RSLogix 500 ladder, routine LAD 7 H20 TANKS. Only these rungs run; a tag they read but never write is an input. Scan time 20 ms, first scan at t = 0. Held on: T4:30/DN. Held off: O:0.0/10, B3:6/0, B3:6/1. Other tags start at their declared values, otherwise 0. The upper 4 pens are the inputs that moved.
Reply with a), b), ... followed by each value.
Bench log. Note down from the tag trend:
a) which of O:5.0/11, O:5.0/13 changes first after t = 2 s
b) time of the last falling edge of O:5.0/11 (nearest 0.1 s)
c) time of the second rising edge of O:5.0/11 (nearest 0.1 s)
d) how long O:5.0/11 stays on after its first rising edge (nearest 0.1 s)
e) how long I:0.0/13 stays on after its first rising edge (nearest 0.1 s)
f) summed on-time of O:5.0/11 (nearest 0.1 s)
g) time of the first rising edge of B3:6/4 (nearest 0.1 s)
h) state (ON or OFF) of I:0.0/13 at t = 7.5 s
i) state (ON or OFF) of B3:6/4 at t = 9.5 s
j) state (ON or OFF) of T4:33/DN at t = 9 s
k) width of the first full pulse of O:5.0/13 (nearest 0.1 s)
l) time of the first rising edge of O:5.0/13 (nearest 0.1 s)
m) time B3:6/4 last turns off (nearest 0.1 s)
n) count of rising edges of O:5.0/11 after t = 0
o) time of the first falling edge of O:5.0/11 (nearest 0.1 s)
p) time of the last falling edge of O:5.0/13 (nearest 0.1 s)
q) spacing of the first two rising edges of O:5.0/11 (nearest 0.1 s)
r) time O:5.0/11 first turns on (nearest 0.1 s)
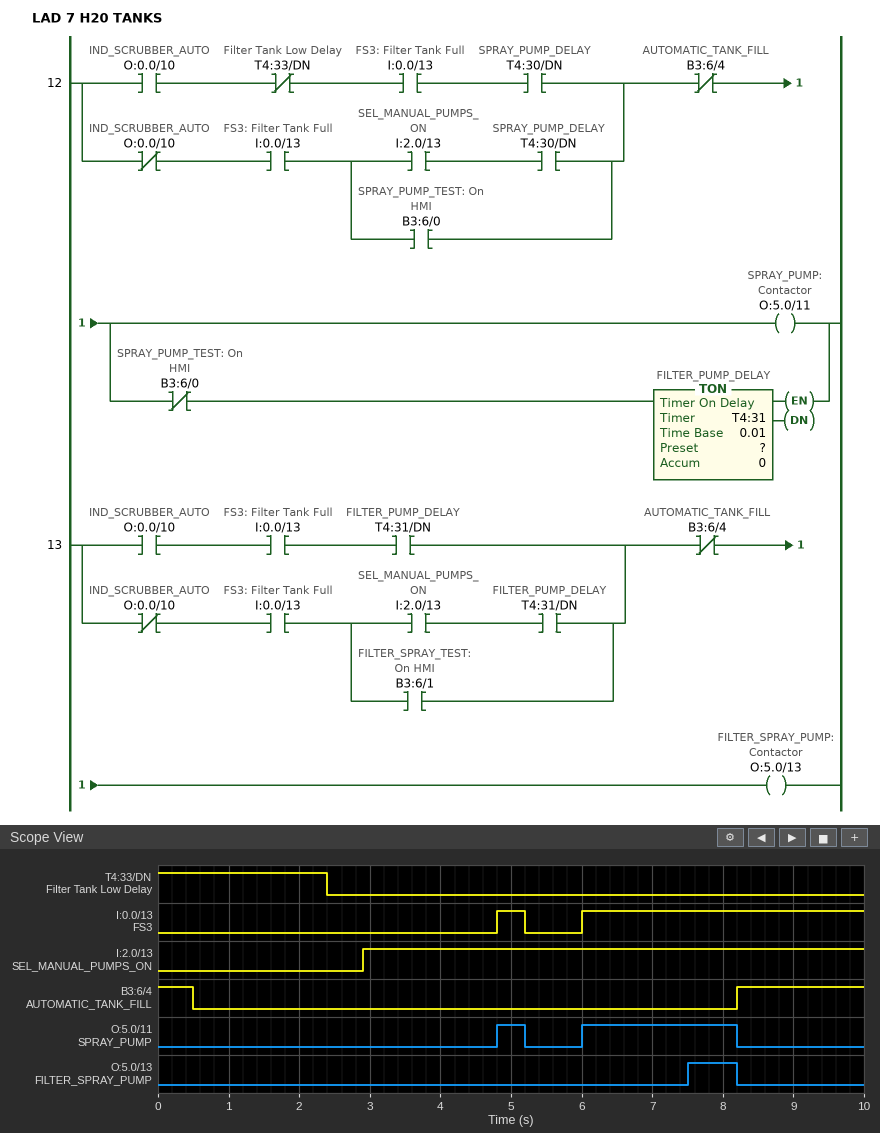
a) O:5.0/11
b) 8.2 s
c) 6.0 s
d) 0.4 s
e) 0.4 s
f) 2.6 s
g) 8.2 s
h) ON
i) ON
j) OFF
k) 0.7 s
l) 7.5 s
m) 0.5 s
n) 2
o) 5.2 s
p) 8.2 s
q) 1.2 s
r) 4.8 s
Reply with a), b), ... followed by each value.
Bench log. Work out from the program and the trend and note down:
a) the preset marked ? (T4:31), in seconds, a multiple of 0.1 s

a) 1.5 s
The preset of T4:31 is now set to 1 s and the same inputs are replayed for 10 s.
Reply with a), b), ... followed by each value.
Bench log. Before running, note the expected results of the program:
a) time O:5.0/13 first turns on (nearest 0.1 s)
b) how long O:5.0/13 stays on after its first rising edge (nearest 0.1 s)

a) 7.0 s
b) 1.2 s
